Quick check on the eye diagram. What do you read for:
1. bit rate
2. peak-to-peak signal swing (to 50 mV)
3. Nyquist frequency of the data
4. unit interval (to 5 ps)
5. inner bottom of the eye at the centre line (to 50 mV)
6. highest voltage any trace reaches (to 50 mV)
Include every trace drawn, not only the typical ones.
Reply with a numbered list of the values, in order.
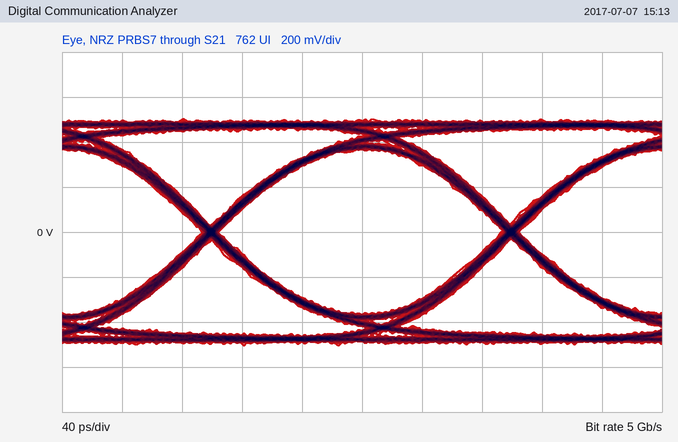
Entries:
1. 5 Gb/s
2. 1.00 V
3. 2.5 GHz
4. 200 ps
5. -350 mV
6. 500 mV
